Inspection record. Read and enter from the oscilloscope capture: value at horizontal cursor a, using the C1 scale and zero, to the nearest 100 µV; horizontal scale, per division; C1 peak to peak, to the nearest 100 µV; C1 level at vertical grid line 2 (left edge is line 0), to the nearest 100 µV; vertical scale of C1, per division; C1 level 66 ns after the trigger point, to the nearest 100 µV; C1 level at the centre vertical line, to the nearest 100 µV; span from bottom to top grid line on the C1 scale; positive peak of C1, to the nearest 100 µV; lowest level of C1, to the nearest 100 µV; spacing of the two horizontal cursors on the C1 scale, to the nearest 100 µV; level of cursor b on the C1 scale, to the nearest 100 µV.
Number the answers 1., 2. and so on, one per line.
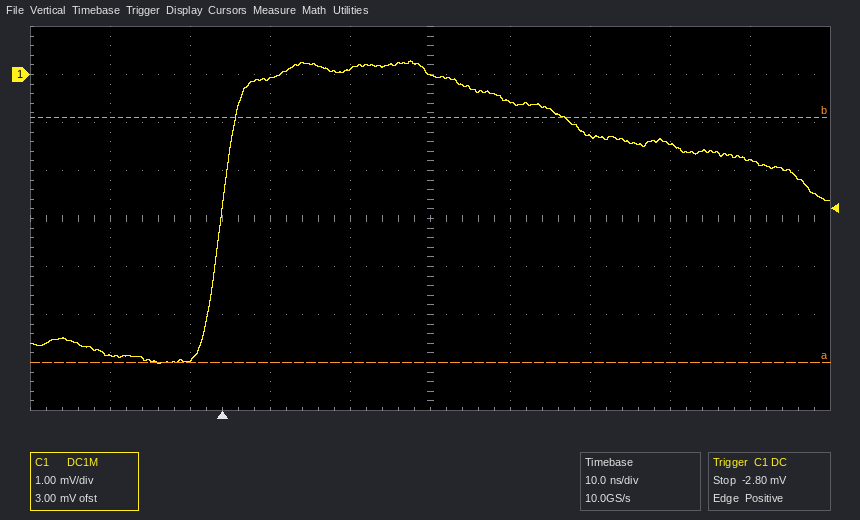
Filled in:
1. -6.0 mV
2. 10 ns
3. 6.3 mV
4. -5.9 mV
5. 1 mV
6. -1.8 mV
7. 0.0 mV
8. 8 mV
9. 300 µV
10. -6.0 mV
11. 5.1 mV
12. -900 µV
